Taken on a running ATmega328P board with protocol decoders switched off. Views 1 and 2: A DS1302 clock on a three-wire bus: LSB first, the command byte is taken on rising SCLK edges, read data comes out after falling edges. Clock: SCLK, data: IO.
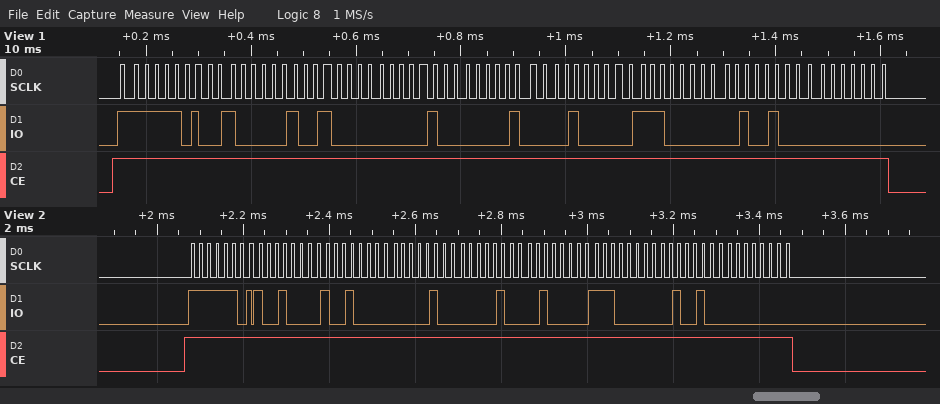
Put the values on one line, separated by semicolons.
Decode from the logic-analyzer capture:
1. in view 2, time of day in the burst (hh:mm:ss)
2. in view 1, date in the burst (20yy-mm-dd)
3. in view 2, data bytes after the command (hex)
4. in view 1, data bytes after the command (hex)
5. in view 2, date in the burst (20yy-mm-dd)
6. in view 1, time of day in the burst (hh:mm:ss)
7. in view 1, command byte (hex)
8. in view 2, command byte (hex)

20:09:09; 2024-04-20; 09 09 20 20 04 07 24 00; 04 09 20 20 04 07 24 00; 2024-04-20; 20:09:04; 0xBF; 0xBF
